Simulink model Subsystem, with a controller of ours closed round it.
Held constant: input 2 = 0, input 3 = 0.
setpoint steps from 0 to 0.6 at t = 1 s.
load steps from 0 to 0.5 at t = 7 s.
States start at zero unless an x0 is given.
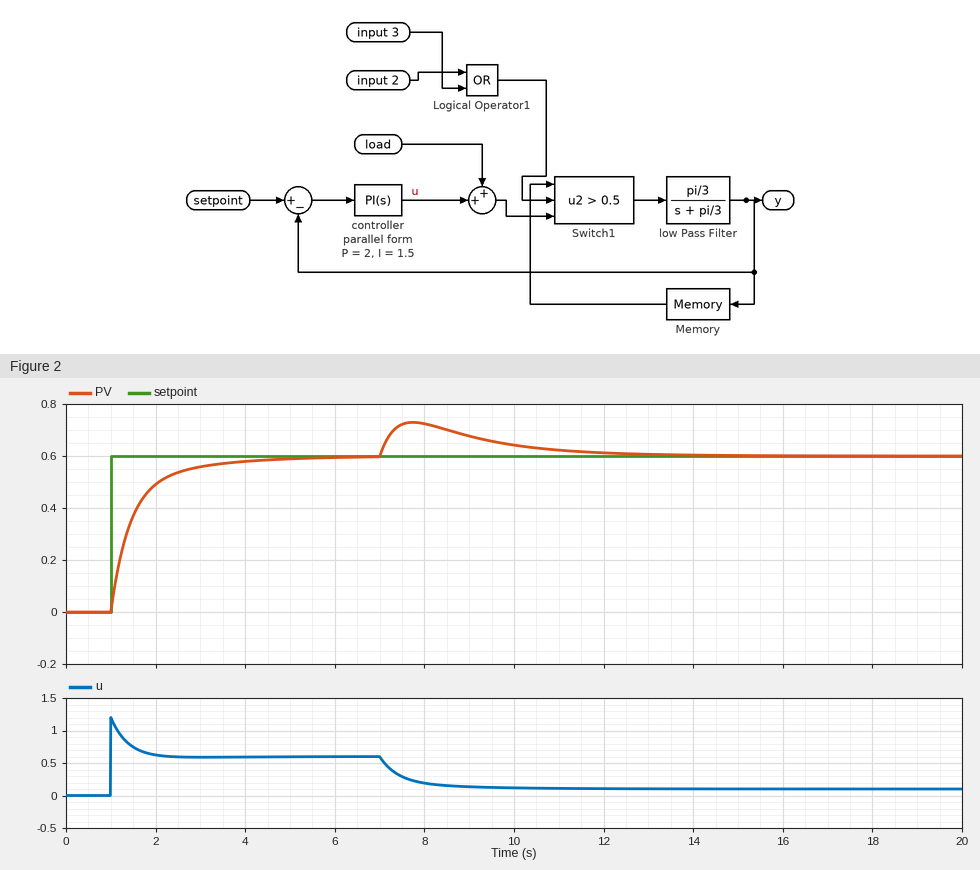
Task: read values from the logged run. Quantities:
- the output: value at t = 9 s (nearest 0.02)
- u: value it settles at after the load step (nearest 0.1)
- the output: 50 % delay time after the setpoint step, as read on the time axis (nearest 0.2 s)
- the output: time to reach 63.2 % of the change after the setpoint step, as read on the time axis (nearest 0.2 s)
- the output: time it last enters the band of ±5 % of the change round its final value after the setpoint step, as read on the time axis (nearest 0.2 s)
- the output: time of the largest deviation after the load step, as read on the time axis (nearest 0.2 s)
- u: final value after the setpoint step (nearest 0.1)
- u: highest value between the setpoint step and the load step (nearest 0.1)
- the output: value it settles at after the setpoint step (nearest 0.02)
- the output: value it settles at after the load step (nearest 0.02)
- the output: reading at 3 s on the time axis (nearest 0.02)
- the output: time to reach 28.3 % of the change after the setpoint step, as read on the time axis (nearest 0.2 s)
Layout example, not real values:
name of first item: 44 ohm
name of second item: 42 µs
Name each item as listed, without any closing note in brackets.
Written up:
the output: value at t = 9 s: 0.68
u: value it settles at after the load step: 0.1
the output: 50 % delay time after the setpoint step, as read on the time axis: 1.4 s
the output: time to reach 63.2 % of the change after the setpoint step, as read on the time axis: 1.6 s
the output: time it last enters the band of ±5 % of the change round its final value after the setpoint step, as read on the time axis: 3.4 s
the output: time of the largest deviation after the load step, as read on the time axis: 7.8 s
u: final value after the setpoint step: 0.6
u: highest value between the setpoint step and the load step: 1.2
the output: value it settles at after the setpoint step: 0.60
the output: value it settles at after the load step: 0.60
the output: reading at 3 s on the time axis: 0.56
the output: time to reach 28.3 % of the change after the setpoint step, as read on the time axis: 1.2 s
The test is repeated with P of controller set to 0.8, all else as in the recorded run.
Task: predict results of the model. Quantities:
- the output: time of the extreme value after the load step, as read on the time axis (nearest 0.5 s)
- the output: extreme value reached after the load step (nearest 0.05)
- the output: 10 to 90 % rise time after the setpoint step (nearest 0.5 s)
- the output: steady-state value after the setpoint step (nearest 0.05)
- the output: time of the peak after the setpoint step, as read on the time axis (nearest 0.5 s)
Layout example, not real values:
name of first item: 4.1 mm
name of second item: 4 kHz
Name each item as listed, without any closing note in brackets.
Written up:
the output: time of the extreme value after the load step, as read on the time axis: 8.0 s
the output: extreme value reached after the load step: 0.80
the output: 10 to 90 % rise time after the setpoint step: 1.5 s
the output: steady-state value after the setpoint step: 0.60
the output: time of the peak after the setpoint step, as read on the time axis: 4.0 s
